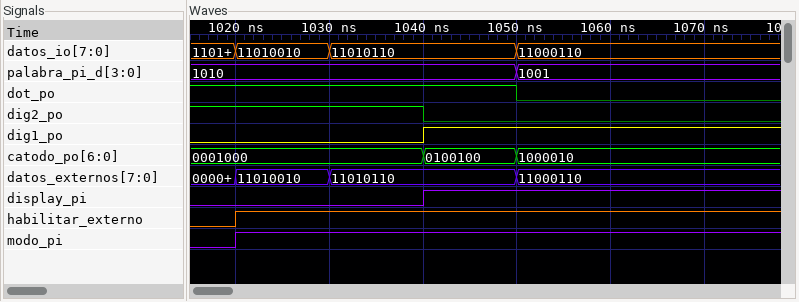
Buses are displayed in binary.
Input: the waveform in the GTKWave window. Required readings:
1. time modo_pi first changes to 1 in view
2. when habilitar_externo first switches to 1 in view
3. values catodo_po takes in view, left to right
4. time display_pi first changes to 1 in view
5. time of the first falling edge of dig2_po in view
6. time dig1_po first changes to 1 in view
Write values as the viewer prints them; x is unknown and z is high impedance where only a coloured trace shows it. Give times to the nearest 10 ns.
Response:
1020 ns
1020 ns
0001000, 0100100, 1000010
1040 ns
1040 ns
1040 ns
